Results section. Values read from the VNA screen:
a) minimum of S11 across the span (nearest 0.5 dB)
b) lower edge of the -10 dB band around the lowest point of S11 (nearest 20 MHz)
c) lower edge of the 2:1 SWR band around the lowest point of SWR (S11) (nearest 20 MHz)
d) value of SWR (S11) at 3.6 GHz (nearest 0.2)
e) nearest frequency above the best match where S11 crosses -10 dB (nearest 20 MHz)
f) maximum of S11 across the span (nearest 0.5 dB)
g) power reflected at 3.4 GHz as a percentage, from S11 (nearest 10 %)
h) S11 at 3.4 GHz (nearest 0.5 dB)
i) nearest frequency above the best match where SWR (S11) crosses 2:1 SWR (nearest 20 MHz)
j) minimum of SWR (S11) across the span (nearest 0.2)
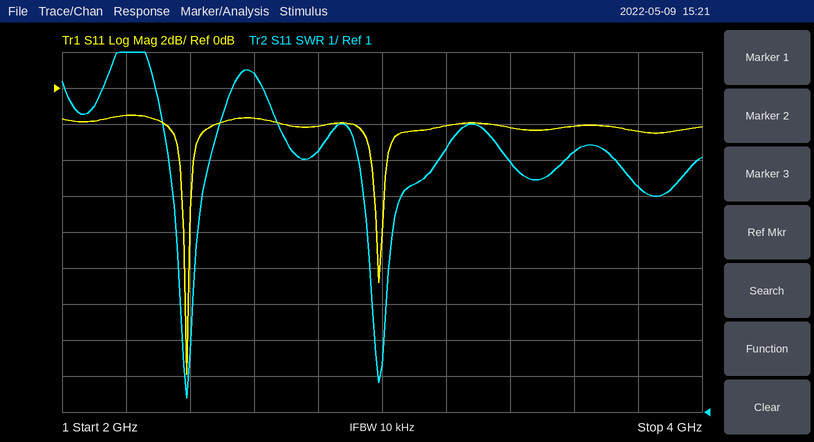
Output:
-16.0 dB
2.38 GHz
2.38 GHz
8.2
2.40 GHz
-1.5 dB
60 %
-2.0 dB
2.40 GHz
1.4
